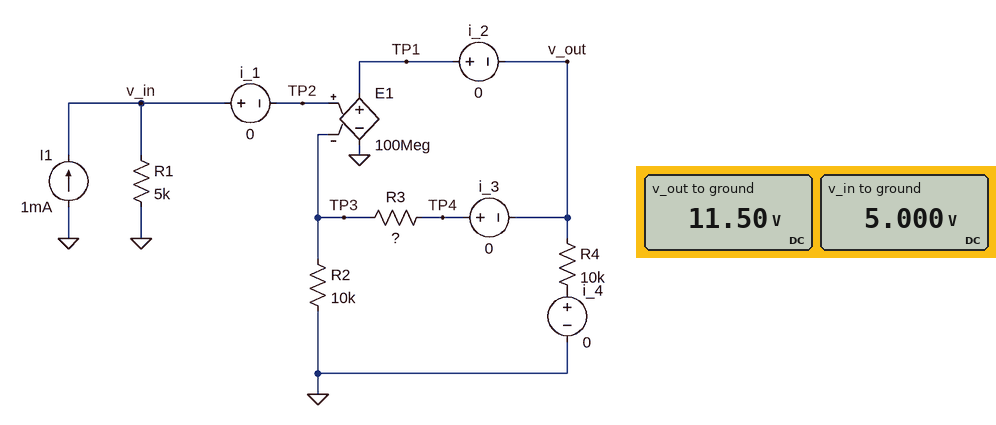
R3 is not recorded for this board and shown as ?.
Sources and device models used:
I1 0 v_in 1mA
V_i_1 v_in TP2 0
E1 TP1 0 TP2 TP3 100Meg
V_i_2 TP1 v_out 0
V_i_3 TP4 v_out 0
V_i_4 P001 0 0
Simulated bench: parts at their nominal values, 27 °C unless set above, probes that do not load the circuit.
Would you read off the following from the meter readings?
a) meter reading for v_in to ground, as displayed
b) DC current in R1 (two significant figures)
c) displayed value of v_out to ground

5.000 V
1.0 mA
11.50 V
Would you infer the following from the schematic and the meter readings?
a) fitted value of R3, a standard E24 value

13 kΩ
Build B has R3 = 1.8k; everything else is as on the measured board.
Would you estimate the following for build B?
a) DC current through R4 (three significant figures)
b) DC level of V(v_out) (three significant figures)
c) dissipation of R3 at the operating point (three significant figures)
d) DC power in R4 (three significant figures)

590 µA
5.90 V
450 µW
3.48 mW
